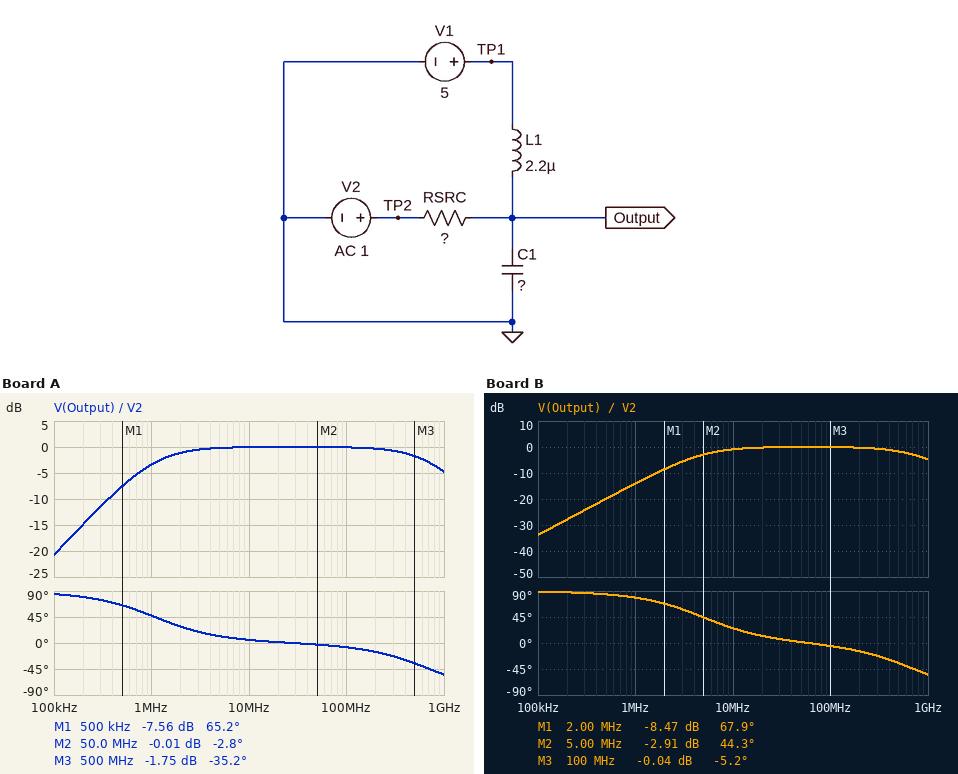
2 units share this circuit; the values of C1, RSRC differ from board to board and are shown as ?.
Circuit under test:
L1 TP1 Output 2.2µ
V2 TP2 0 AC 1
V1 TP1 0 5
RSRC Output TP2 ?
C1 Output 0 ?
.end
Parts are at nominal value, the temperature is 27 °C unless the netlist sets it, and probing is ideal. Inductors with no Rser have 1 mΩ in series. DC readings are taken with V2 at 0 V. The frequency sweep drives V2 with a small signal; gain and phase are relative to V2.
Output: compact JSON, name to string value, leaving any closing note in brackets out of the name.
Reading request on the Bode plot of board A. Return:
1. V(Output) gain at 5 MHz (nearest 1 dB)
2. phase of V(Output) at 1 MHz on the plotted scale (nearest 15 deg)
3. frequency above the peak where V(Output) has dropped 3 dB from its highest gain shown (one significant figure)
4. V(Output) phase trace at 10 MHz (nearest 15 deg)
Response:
{"V(Output) gain at 5 MHz": "0 dB", "phase of V(Output) at 1 MHz on the plotted scale": "45 deg", "frequency above the peak where V(Output) has dropped 3 dB from its highest gain shown": "700 MHz", "V(Output) phase trace at 10 MHz": "0 deg"}
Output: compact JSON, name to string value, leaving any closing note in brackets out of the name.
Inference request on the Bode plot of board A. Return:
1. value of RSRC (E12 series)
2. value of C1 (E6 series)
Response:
{"value of RSRC": "15 Ω", "value of C1": "15 pF"}
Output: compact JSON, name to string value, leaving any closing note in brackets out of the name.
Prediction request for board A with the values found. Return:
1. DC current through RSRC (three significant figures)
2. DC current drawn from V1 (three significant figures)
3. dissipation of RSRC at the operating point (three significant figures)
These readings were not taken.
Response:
{"DC current through RSRC": "333 mA", "DC current drawn from V1": "333 mA", "dissipation of RSRC at the operating point": "1.67 W"}
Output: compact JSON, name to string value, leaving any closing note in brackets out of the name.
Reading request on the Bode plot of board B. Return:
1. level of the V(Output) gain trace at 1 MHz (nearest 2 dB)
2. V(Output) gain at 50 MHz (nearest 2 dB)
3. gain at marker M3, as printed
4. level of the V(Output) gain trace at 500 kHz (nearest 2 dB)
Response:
{"level of the V(Output) gain trace at 1 MHz": "-14 dB", "V(Output) gain at 50 MHz": "0 dB", "gain at marker M3, as printed": "-0.04 dB", "level of the V(Output) gain trace at 500 kHz": "-20 dB"}
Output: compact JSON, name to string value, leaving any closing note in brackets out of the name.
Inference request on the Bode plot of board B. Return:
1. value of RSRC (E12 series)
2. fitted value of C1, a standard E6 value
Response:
{"value of RSRC": "68 Ω", "fitted value of C1, a standard E6 value": "3.3 pF"}
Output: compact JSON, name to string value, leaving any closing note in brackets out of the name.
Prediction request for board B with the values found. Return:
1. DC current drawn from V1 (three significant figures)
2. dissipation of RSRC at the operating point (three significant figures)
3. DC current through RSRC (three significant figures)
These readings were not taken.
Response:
{"DC current drawn from V1": "73.5 mA", "dissipation of RSRC at the operating point": "368 mW", "DC current through RSRC": "73.5 mA"}
